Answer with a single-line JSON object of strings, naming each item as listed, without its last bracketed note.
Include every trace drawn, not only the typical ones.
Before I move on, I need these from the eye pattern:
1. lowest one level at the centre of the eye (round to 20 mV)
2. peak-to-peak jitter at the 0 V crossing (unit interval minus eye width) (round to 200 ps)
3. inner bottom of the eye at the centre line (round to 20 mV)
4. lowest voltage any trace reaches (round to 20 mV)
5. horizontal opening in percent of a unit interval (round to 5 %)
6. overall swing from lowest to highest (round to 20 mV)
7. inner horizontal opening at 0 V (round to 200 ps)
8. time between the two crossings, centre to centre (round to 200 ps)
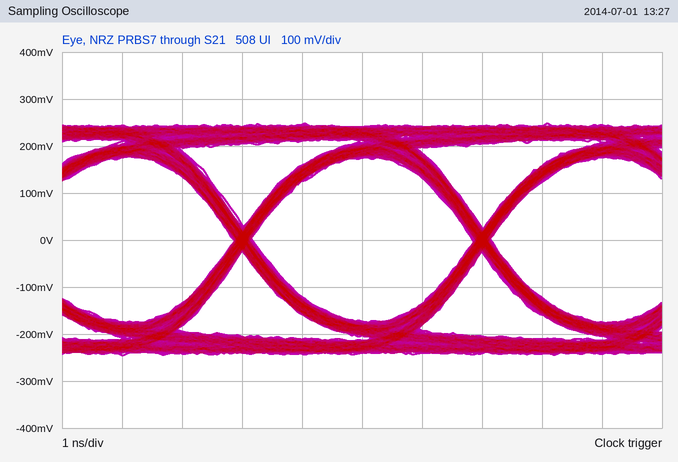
{"lowest one level at the centre of the eye": "180 mV", "peak-to-peak jitter at the 0 V crossing (unit interval minus eye width)": "400 ps", "inner bottom of the eye at the centre line": "-180 mV", "lowest voltage any trace reaches": "-240 mV", "horizontal opening in percent of a unit interval": "90 %", "overall swing from lowest to highest": "500 mV", "inner horizontal opening at 0 V": "3.6 ns", "time between the two crossings, centre to centre": "4.0 ns"}
